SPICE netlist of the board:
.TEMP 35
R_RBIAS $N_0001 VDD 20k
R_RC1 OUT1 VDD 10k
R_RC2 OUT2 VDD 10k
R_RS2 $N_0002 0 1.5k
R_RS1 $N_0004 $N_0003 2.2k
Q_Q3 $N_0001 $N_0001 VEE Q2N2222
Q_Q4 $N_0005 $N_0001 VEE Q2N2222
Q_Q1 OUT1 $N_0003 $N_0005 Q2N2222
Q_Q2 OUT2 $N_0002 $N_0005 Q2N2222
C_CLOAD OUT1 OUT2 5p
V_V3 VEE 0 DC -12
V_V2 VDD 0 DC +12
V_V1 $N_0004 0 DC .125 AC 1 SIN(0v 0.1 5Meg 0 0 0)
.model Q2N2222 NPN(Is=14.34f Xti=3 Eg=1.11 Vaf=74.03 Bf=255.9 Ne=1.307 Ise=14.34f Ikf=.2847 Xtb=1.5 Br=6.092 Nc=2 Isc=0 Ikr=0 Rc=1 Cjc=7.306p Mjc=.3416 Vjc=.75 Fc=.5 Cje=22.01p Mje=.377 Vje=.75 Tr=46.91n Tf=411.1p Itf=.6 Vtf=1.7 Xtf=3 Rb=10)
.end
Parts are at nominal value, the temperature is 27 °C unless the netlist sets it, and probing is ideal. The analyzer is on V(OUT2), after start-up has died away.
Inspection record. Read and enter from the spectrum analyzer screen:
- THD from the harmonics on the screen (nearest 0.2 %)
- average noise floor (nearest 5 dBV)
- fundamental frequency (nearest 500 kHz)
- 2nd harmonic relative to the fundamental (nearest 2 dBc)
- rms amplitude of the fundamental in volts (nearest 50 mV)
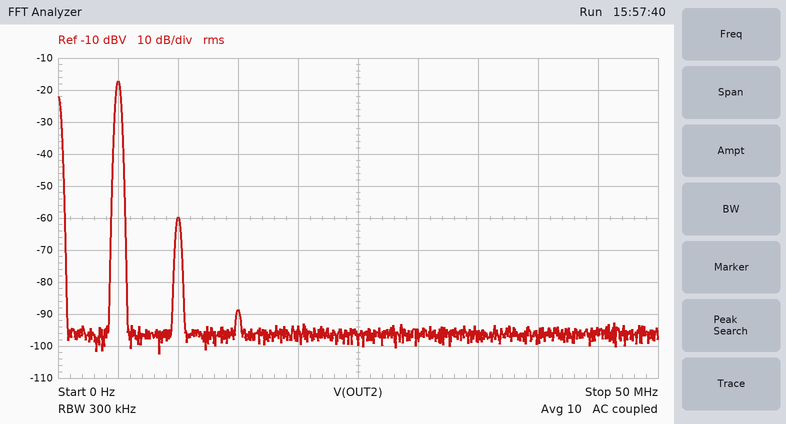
0.8 %
-95 dBV
5.0 MHz
-42 dBc
150 mV
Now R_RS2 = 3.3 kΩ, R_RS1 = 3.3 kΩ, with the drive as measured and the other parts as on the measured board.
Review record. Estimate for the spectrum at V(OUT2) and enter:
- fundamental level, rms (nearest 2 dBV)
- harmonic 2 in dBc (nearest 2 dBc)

-22 dBV
-50 dBc
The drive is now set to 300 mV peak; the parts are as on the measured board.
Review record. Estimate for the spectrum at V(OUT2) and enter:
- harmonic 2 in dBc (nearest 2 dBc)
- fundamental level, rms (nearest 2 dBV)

-32 dBc
-8 dBV
